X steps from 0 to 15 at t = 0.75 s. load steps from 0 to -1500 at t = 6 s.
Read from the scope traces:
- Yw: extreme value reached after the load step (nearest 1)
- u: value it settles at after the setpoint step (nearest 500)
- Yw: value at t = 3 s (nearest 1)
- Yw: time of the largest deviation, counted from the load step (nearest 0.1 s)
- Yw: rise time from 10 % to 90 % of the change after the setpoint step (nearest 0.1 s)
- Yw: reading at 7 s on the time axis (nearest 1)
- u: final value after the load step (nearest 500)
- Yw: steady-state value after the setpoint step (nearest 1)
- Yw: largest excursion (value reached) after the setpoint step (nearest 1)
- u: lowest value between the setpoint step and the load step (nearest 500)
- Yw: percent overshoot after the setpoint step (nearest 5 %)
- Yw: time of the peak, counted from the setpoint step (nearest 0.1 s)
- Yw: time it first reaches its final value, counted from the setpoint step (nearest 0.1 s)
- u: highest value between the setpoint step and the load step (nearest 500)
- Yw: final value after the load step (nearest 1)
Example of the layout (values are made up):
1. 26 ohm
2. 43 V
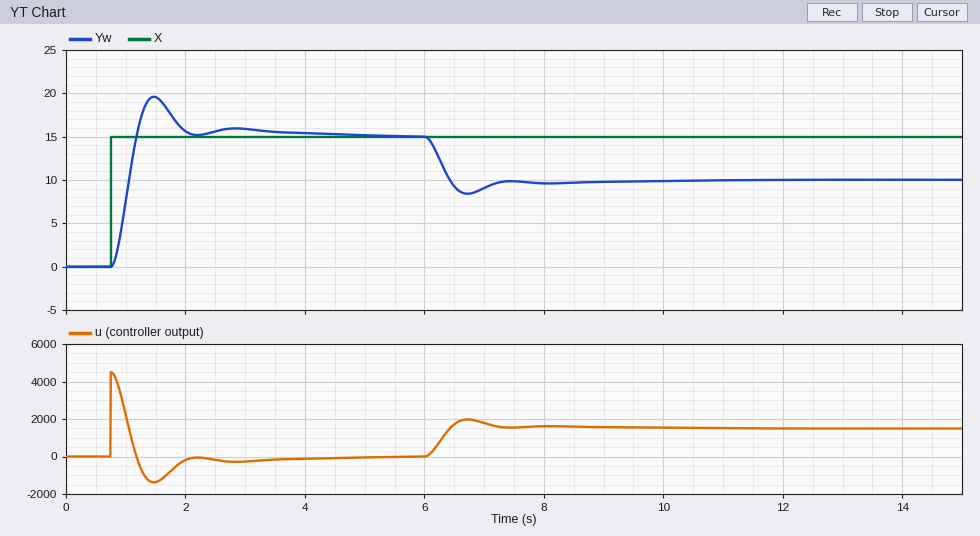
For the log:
1. 8
2. 0
3. 16
4. 0.7 s
5. 0.3 s
6. 9
7. 1500
8. 15
9. 20
10. -1500
11. 30 %
12. 0.7 s
13. 0.4 s
14. 4500
15. 10
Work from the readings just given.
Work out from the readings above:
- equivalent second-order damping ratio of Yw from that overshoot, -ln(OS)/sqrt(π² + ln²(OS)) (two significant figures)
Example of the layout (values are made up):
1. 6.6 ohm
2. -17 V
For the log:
1. 0.36
